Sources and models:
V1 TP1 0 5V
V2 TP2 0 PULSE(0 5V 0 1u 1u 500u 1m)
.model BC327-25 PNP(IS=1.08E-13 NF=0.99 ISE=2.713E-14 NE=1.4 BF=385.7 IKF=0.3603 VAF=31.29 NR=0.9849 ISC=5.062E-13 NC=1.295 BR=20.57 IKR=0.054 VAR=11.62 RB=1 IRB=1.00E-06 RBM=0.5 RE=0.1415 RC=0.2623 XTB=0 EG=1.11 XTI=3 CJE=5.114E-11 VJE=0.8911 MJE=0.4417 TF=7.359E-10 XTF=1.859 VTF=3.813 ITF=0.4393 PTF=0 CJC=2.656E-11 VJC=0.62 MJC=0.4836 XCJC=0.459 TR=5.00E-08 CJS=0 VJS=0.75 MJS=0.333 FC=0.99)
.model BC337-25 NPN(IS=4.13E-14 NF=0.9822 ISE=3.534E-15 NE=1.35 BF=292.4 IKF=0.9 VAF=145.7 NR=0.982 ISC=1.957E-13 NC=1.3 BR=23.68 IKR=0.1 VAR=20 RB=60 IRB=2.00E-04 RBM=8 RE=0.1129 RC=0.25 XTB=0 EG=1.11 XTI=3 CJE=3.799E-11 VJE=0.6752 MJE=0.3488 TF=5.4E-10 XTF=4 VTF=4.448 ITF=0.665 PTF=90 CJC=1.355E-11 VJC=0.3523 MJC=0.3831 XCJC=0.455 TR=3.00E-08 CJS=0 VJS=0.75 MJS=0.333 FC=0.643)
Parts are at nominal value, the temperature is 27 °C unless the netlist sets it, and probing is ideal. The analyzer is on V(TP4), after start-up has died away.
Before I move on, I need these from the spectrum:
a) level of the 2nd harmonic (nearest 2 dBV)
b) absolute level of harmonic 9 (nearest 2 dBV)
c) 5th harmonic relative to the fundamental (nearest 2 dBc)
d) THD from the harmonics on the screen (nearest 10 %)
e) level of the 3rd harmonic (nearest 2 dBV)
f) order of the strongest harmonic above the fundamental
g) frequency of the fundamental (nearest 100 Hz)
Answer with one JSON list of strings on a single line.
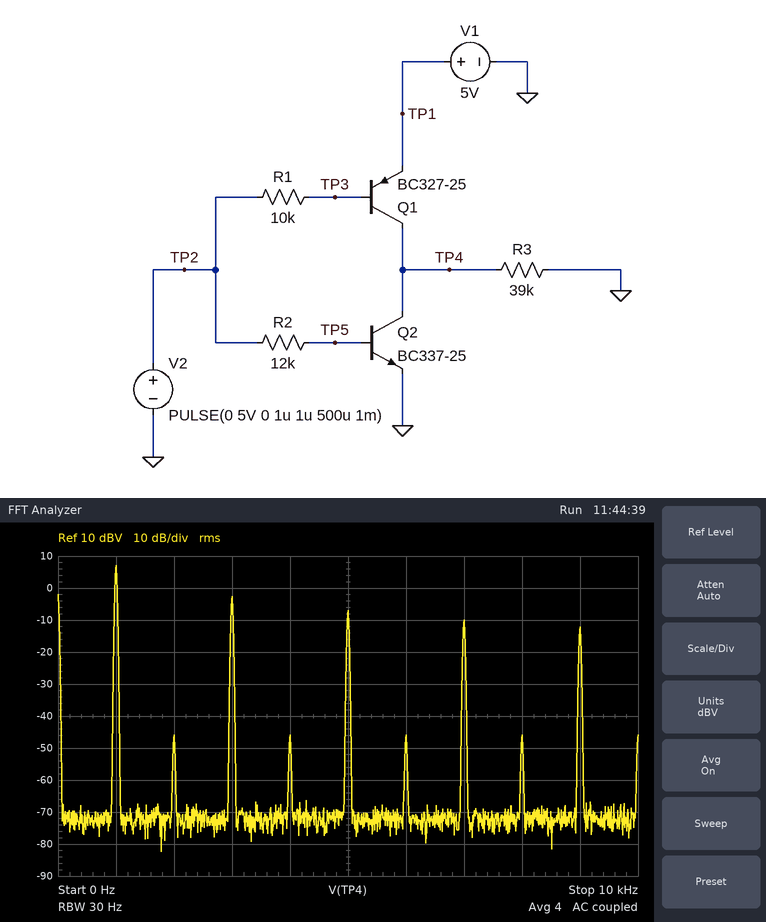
["-46 dBV", "-12 dBV", "-14 dBc", "40 %", "-2 dBV", "3", "1.0 kHz"]
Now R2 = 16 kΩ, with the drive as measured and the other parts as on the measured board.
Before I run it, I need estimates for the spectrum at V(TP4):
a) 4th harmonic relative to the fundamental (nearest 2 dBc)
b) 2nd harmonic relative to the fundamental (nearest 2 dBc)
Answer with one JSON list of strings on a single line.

["-56 dBc", "-56 dBc"]
